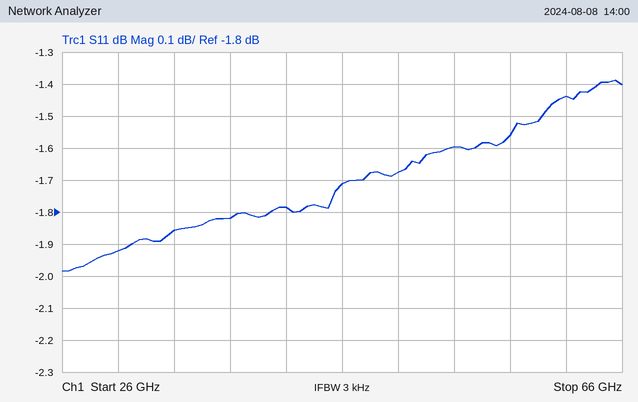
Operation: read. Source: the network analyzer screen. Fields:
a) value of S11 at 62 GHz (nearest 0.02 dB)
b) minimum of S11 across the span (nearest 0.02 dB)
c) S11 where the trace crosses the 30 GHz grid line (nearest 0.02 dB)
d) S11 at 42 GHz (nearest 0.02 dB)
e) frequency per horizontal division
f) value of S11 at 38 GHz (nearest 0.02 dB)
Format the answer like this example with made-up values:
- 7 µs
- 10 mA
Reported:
- -1.44 dB
- -1.98 dB
- -1.92 dB
- -1.78 dB
- 4 GHz
- -1.82 dB
